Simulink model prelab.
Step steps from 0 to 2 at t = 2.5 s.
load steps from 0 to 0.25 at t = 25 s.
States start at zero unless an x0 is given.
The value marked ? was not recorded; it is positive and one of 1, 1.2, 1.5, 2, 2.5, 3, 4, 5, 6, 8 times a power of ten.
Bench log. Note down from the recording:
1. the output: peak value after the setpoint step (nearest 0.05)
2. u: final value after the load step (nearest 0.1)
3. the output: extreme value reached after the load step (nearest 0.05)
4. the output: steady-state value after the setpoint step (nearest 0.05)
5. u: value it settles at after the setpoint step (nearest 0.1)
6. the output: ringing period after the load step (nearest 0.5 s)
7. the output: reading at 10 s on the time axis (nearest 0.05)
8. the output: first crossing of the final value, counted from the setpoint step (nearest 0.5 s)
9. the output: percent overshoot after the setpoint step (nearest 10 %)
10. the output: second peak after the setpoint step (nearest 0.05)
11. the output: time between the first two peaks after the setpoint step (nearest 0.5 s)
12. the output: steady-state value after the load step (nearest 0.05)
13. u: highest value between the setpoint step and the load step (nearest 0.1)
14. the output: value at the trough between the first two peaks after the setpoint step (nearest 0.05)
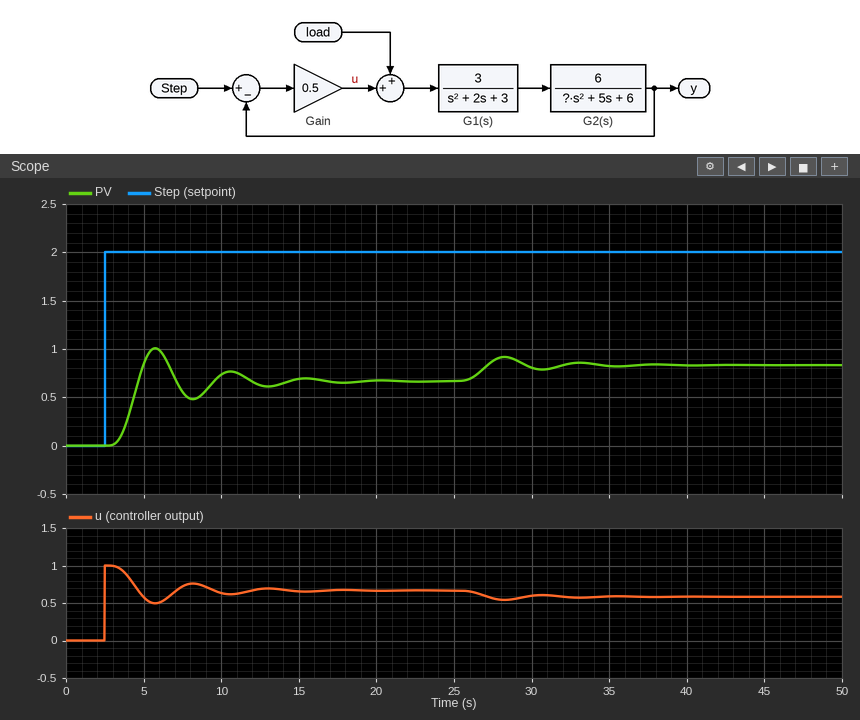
1.00
0.6
0.90
0.65
0.7
5.0 s
0.75
2.0 s
50 %
0.75
5.0 s
0.85
1.0
0.50
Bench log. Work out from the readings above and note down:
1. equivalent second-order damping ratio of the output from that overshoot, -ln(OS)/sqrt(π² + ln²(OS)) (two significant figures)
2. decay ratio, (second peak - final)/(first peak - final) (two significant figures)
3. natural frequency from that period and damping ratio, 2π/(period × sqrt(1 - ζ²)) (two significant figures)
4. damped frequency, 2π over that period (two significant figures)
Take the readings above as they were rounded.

0.22
0.29
1.3 rad/s
1.3 rad/s
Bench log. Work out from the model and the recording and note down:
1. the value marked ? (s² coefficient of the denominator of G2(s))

4
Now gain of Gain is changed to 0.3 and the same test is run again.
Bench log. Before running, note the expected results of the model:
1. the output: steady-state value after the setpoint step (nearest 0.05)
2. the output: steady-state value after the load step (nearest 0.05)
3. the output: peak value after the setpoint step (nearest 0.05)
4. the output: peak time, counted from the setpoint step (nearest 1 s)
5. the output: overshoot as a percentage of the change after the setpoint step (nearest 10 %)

0.45
0.65
0.65
3 s
40 %
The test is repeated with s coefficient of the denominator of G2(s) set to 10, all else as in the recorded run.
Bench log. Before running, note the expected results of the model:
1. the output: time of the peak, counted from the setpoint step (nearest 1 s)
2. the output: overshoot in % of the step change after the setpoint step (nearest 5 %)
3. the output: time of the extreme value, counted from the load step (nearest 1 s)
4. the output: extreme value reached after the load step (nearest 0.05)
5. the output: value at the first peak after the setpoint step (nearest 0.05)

4 s
15 %
4 s
0.85
0.75
